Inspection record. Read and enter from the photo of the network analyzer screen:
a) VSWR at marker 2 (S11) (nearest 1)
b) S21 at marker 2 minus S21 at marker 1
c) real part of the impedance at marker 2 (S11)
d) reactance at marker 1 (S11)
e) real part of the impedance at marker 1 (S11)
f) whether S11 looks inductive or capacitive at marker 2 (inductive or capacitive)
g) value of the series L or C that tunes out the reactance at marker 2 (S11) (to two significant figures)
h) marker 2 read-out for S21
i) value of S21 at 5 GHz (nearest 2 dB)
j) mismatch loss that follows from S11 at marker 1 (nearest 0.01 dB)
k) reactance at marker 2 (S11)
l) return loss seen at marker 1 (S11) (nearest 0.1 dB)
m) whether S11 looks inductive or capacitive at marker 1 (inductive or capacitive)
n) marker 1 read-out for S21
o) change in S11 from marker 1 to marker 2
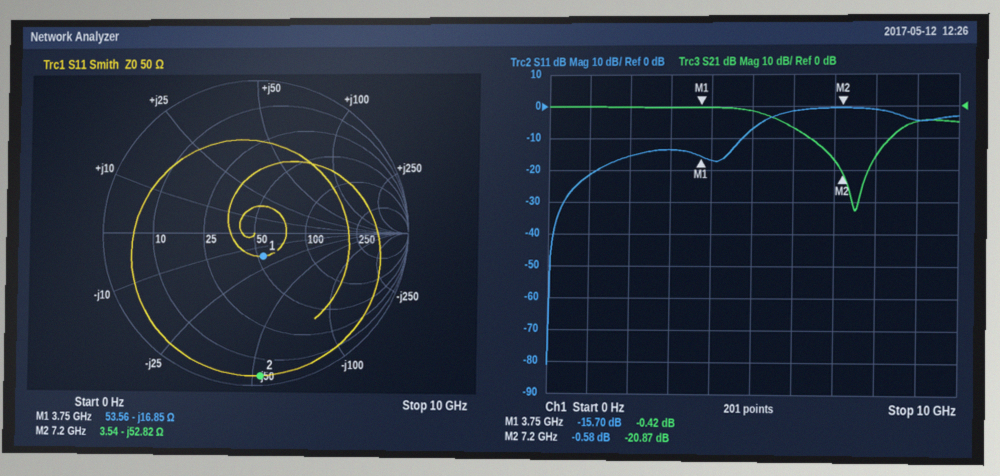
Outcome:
30
-20.45 dB
3.54 Ω
-16.85 Ω
53.56 Ω
capacitive
1.2 nH
-20.87 dB
-2 dB
0.12 dB
-52.82 Ω
15.7 dB
capacitive
-0.42 dB
15.12 dB
